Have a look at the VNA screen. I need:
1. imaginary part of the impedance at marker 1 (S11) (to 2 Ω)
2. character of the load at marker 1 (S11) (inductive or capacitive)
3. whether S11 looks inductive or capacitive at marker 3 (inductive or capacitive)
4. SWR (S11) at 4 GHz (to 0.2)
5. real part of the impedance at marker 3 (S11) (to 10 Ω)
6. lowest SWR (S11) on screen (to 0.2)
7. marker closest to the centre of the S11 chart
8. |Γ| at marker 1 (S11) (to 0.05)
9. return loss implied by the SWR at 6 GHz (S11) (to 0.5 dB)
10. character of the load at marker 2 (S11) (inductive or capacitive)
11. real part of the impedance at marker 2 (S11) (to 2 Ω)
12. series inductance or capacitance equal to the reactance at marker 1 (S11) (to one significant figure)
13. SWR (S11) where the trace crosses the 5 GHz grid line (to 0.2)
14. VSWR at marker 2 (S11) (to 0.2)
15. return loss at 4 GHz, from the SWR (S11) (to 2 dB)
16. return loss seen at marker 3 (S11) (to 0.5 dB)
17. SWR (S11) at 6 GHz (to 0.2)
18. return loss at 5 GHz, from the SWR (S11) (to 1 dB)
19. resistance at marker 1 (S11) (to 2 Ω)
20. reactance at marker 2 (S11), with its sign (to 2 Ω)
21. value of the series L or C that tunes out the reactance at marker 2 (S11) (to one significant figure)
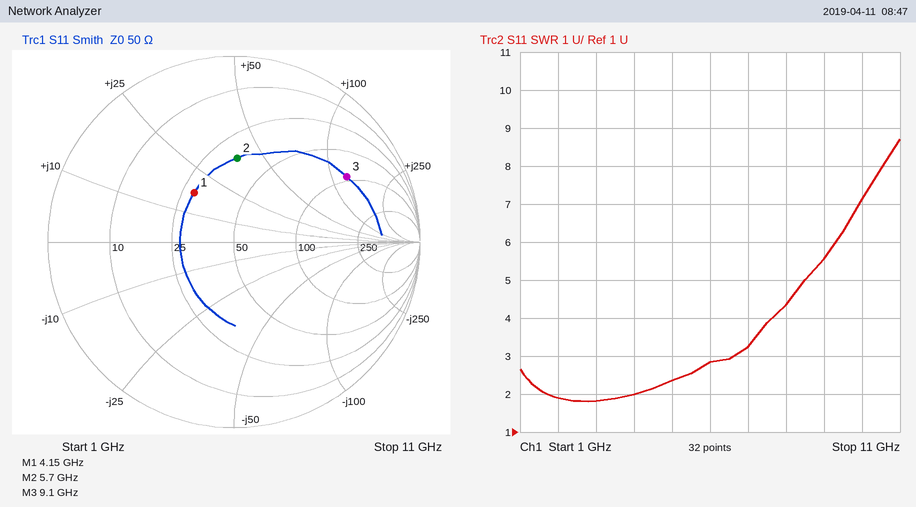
+18 Ω
inductive
inductive
2.0
90 Ω
1.8
marker 1
0.35
6.5 dB
inductive
34 Ω
700 pH
2.4
2.6
10 dB
3.0 dB
2.8
8 dB
28 Ω
+38 Ω
700 fF
